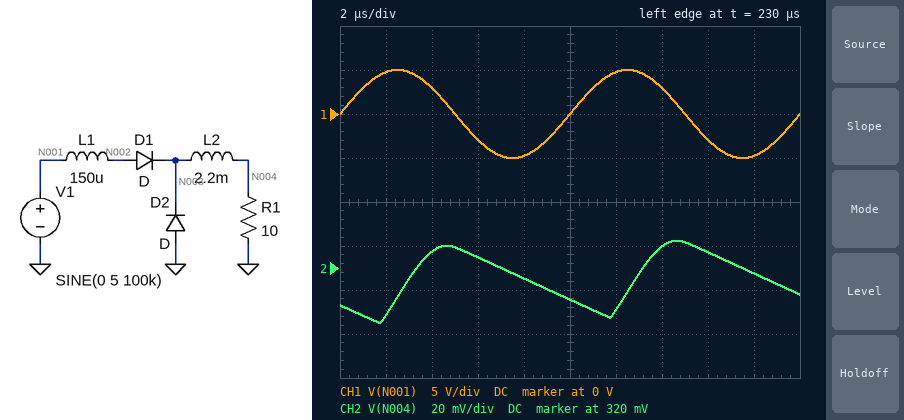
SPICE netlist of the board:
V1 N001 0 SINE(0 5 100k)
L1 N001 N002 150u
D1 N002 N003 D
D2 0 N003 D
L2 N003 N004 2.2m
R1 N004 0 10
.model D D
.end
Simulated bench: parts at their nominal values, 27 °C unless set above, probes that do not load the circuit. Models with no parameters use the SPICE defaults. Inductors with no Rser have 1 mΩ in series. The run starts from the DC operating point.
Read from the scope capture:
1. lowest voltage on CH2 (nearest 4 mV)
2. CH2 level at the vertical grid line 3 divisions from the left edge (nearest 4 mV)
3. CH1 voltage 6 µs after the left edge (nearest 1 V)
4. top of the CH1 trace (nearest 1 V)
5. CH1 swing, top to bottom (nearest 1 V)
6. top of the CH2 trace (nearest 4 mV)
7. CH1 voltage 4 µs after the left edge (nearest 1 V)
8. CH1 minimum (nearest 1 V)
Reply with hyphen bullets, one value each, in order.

- 296 mV
- 324 mV
- -3 V
- 5 V
- 10 V
- 332 mV
- 3 V
- -5 V
